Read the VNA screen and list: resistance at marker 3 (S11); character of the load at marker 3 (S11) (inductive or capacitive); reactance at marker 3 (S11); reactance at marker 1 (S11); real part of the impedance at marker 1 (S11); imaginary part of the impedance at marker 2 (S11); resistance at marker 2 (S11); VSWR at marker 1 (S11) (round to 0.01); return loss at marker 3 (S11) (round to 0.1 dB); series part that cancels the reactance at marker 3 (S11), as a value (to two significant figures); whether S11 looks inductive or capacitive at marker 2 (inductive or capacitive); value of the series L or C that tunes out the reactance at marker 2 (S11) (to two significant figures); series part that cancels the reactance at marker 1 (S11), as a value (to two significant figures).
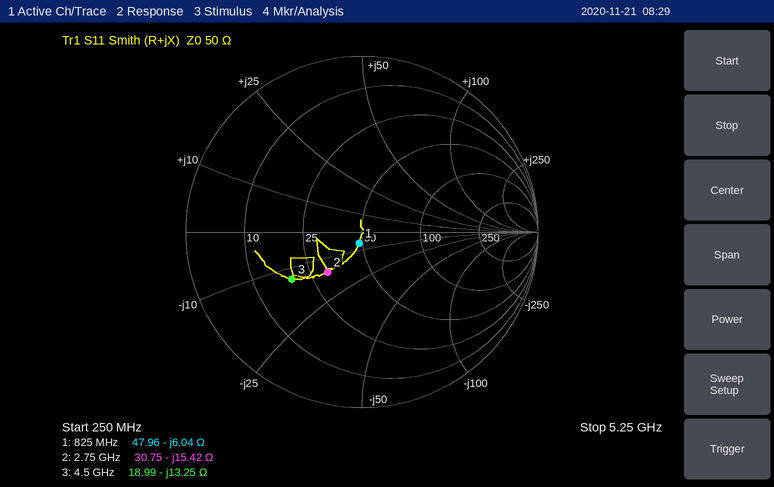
18.99 Ω
capacitive
-13.25 Ω
-6.04 Ω
47.96 Ω
-15.42 Ω
30.75 Ω
1.14
6.4 dB
470 pH
capacitive
890 pH
1.2 nH
